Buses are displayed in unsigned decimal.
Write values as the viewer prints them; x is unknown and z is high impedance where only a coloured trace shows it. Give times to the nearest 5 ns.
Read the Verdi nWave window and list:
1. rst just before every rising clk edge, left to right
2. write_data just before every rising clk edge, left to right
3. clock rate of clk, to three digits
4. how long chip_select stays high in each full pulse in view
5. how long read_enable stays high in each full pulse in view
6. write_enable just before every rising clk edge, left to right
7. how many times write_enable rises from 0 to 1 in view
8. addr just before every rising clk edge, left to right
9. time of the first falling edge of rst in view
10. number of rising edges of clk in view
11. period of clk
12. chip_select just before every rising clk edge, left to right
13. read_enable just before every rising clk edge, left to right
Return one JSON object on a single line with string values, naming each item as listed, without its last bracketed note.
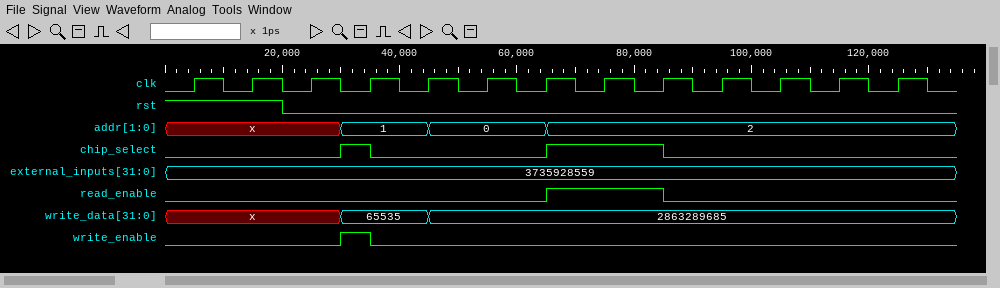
{"rst just before every rising clk edge, left to right": "1 1 0 0 0 0 0 0 0 0 0 0 0", "write_data just before every rising clk edge, left to right": "x, x, x, 65535, 65535, 2863289685, 2863289685, 2863289685, 2863289685, 2863289685, 2863289685, 2863289685, 2863289685", "clock rate of clk, to three digits": "100 MHz", "how long chip_select stays high in each full pulse in view": "5 ns, 20 ns", "how long read_enable stays high in each full pulse in view": "20 ns", "write_enable just before every rising clk edge, left to right": "0 0 0 1 0 0 0 0 0 0 0 0 0", "how many times write_enable rises from 0 to 1 in view": "1", "addr just before every rising clk edge, left to right": "x, x, x, 1, 1, 0, 0, 2, 2, 2, 2, 2, 2", "time of the first falling edge of rst in view": "20 ns", "number of rising edges of clk in view": "13", "period of clk": "10 ns", "chip_select just before every rising clk edge, left to right": "0 0 0 1 0 0 0 1 1 0 0 0 0", "read_enable just before every rising clk edge, left to right": "0 0 0 0 0 0 0 1 1 0 0 0 0"}
